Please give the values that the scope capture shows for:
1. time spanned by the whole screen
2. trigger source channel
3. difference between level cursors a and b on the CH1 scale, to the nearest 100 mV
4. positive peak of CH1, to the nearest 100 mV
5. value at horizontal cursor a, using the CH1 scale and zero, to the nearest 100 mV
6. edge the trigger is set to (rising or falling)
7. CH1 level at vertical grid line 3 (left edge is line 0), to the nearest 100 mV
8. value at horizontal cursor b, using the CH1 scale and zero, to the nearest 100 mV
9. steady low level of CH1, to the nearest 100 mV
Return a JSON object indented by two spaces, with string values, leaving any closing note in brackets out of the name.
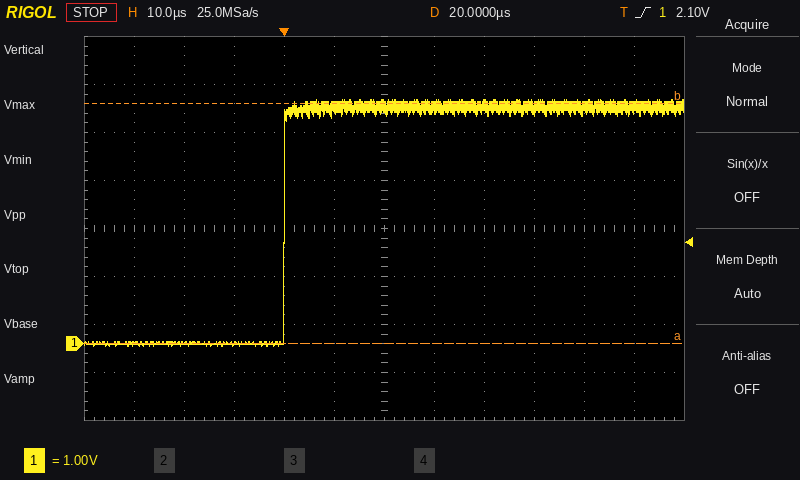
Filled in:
{
  "time spanned by the whole screen": "120 µs",
  "trigger source channel": "CH1",
  "difference between level cursors a and b on the CH1 scale, to the nearest 100 mV": "5.0 V",
  "positive peak of CH1, to the nearest 100 mV": "5.1 V",
  "value at horizontal cursor a, using the CH1 scale and zero, to the nearest 100 mV": "0.0 V",
  "edge the trigger is set to": "rising",
  "CH1 level at vertical grid line 3 (left edge is line 0), to the nearest 100 mV": "0.0 V",
  "value at horizontal cursor b, using the CH1 scale and zero, to the nearest 100 mV": "5.0 V",
  "steady low level of CH1, to the nearest 100 mV": "0.0 V"
}
